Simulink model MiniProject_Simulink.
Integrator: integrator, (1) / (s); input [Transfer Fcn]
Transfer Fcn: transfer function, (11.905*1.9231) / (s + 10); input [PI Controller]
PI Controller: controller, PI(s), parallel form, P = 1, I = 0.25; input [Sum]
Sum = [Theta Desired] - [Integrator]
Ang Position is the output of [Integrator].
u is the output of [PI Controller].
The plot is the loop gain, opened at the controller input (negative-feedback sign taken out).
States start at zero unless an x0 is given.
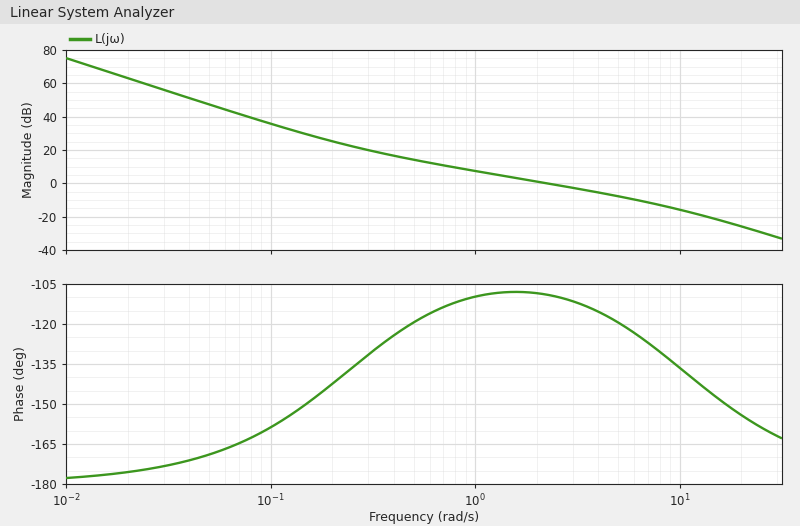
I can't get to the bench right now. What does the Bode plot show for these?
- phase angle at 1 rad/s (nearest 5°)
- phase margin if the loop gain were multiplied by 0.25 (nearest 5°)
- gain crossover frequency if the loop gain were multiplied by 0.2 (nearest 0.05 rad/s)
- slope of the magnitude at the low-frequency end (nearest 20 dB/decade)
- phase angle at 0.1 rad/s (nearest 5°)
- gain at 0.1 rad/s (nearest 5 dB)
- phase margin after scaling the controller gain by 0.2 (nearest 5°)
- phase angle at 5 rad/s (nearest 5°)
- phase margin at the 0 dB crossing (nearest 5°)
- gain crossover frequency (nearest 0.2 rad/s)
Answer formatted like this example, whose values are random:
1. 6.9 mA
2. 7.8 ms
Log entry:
1. -110°
2. 65°
3. 0.50 rad/s
4. -40 dB/decade
5. -160°
6. 35 dB
7. 60°
8. -120°
9. 70°
10. 2.2 rad/s
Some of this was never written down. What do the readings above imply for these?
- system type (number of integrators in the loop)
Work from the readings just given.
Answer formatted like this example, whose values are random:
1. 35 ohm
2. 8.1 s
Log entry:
1. 2
